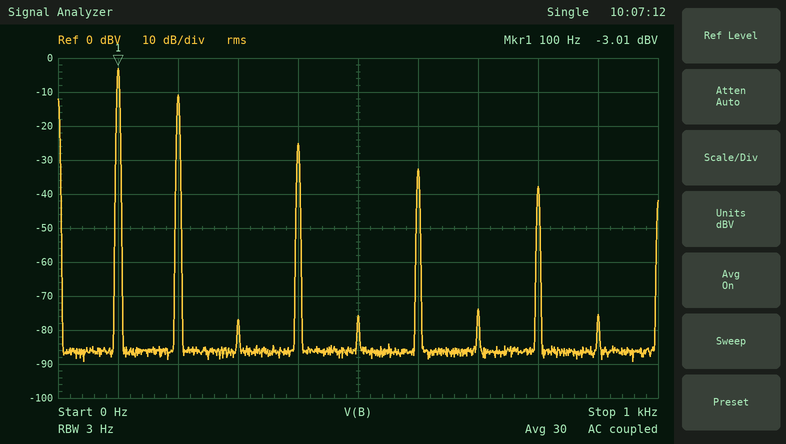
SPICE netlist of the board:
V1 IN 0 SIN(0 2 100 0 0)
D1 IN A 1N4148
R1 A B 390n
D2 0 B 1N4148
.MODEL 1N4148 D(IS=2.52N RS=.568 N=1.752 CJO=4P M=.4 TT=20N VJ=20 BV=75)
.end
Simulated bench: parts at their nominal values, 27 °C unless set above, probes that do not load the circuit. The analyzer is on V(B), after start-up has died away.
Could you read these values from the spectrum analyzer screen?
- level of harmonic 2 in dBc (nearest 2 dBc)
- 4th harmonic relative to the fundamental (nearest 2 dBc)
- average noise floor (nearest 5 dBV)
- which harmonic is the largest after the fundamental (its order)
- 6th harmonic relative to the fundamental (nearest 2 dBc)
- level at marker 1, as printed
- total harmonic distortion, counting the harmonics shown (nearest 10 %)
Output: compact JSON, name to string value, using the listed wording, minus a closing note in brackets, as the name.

{"level of harmonic 2 in dBc": "-8 dBc", "4th harmonic relative to the fundamental": "-22 dBc", "average noise floor": "-85 dBV", "which harmonic is the largest after the fundamental": "2", "6th harmonic relative to the fundamental": "-30 dBc", "level at marker 1, as printed": "-3.01 dBV", "total harmonic distortion, counting the harmonics shown": "40 %"}
